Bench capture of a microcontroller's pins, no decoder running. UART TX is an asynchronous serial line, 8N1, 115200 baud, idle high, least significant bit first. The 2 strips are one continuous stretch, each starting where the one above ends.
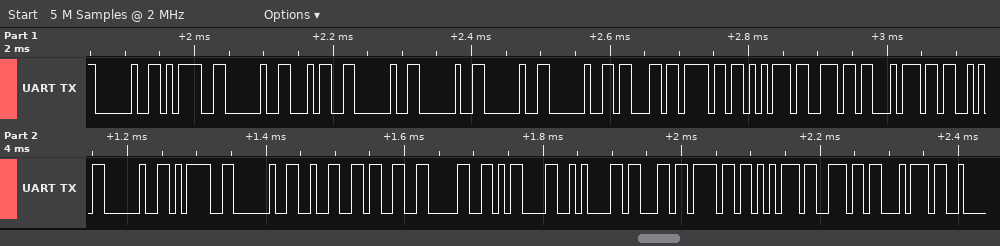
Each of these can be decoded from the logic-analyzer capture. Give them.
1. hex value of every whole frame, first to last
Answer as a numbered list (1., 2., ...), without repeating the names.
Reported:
1. 20 3D 20 34 20 20 20 20 63 6F 75 6E 74 53 20 3D 20 32 33 30 0D 0A 63 6F 75 6E 74
